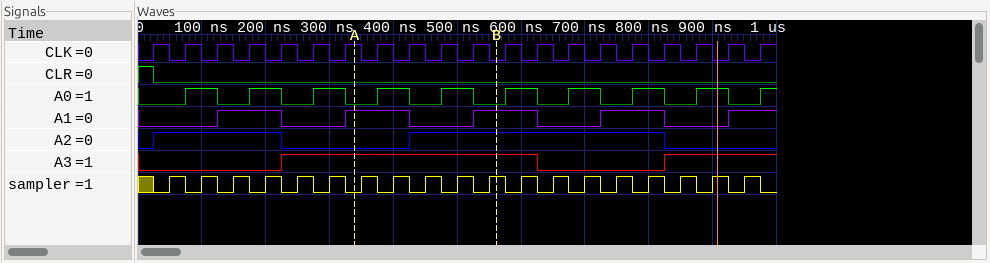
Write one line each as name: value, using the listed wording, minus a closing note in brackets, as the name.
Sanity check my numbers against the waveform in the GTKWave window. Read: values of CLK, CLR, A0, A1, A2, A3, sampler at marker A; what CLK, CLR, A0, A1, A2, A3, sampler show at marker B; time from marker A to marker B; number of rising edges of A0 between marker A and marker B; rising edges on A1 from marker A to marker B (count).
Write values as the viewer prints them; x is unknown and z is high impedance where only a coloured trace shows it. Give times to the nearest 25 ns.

values of CLK, CLR, A0, A1, A2, A3, sampler at marker A: CLK=1, CLR=0, A0=0, A1=1, A2=0, A3=1, sampler=0
what CLK, CLR, A0, A1, A2, A3, sampler show at marker B: CLK=0, CLR=0, A0=0, A1=1, A2=1, A3=1, sampler=1
time from marker A to marker B: 225 ns
number of rising edges of A0 between marker A and marker B: 2
rising edges on A1 from marker A to marker B: 1
